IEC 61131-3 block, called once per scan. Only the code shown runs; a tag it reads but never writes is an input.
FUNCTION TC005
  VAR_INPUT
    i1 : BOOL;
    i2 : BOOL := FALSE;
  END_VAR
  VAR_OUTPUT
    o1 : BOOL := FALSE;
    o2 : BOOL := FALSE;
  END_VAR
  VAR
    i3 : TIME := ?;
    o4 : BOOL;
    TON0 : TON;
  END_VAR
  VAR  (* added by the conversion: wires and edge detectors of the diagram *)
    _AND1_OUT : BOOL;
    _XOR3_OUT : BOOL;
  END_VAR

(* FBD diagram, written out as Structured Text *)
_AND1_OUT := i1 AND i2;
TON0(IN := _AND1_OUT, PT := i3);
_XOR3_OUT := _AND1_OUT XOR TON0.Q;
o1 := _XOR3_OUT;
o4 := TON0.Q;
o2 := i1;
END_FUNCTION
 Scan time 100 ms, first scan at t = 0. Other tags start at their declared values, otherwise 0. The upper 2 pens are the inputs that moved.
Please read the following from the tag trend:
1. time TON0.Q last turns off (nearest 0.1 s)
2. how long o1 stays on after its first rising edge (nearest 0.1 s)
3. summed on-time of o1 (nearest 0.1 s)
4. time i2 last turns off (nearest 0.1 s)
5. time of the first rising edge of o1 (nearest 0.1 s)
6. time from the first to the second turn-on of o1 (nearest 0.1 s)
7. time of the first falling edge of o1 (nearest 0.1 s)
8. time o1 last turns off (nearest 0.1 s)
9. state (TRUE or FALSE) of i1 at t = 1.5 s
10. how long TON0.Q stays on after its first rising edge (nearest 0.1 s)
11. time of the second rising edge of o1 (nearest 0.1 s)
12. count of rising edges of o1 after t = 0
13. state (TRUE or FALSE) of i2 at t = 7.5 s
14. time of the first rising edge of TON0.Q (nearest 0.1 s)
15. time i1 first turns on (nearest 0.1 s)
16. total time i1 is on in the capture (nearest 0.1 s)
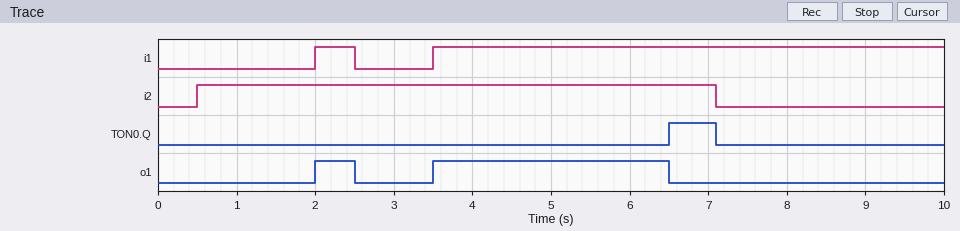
7.1 s
0.5 s
3.5 s
7.1 s
2.0 s
1.5 s
2.5 s
6.5 s
FALSE
0.6 s
3.5 s
2
FALSE
6.5 s
2.0 s
7.0 s
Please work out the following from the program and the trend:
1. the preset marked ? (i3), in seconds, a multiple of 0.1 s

3.0 s
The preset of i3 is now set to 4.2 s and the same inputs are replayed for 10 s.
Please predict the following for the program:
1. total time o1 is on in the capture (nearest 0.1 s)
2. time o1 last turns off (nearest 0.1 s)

4.1 s
7.1 s
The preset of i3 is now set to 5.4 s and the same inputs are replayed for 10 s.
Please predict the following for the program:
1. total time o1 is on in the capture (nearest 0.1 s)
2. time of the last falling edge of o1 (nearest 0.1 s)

4.1 s
7.1 s
